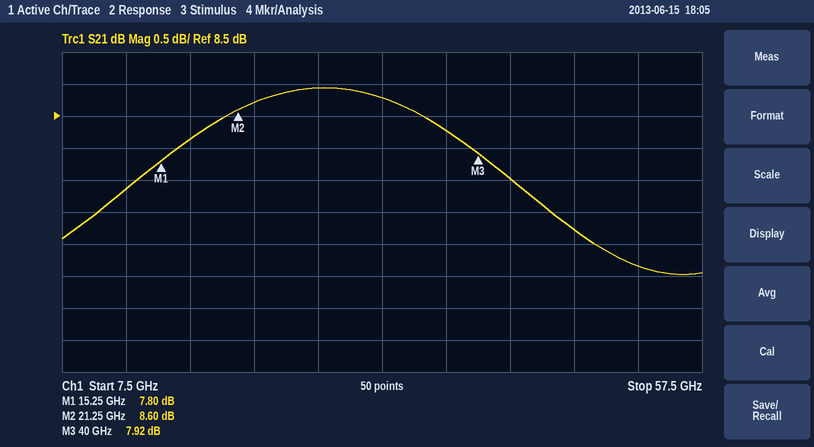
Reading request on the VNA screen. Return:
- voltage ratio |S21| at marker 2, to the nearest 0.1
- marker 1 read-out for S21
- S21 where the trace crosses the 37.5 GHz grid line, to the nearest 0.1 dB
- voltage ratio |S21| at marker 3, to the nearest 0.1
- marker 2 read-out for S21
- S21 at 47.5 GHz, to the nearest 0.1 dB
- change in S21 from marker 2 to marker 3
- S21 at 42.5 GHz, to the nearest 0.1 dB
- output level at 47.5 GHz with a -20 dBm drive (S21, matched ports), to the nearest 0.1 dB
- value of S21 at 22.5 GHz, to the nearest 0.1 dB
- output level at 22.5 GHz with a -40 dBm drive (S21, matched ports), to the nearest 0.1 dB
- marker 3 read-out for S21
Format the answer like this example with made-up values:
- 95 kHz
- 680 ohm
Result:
- 2.7
- 7.80 dB
- 8.3 dB
- 2.5
- 8.60 dB
- 6.7 dB
- -0.68 dB
- 7.5 dB
- -13.3 dBm
- 8.7 dB
- -31.3 dBm
- 7.92 dB
